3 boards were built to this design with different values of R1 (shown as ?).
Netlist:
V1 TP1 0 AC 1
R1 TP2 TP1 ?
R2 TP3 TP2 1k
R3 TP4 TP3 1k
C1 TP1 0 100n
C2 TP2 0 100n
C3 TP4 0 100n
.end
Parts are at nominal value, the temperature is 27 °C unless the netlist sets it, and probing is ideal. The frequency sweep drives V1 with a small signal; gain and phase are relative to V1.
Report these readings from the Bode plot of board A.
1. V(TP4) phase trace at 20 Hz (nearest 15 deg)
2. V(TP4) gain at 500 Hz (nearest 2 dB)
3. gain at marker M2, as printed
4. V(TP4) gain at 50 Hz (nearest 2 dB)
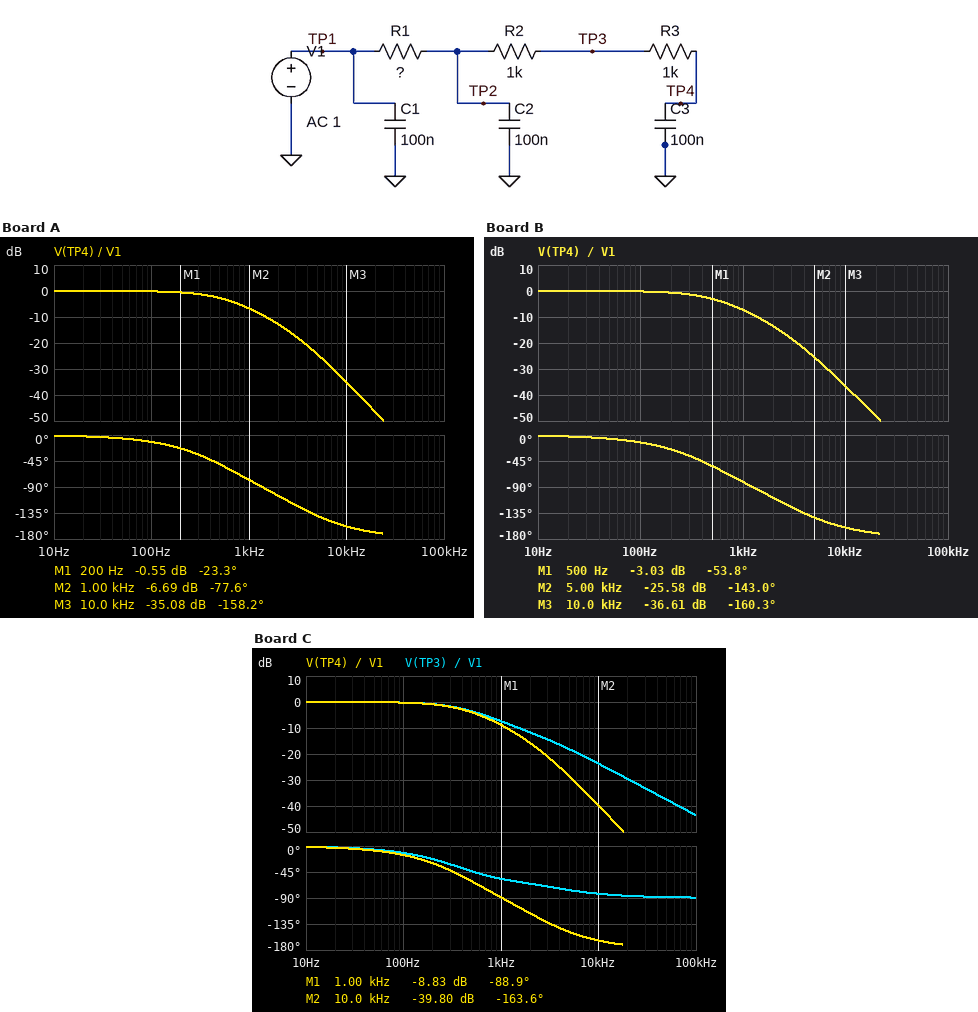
0 deg
-2 dB
-6.69 dB
0 dB
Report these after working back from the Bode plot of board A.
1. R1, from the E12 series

680 Ω
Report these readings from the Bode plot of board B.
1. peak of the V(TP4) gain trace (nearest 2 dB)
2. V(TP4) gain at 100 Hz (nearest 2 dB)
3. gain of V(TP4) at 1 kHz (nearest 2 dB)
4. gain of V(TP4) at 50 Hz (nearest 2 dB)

0 dB
0 dB
-8 dB
0 dB
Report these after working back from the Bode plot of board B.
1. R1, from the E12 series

820 Ω
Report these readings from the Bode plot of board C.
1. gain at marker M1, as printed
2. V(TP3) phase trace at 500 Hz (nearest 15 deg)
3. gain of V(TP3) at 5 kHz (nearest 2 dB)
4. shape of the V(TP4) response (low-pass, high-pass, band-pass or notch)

-8.83 dB
-45 deg
-18 dB
low-pass
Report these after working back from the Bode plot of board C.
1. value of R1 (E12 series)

1.2 kΩ
